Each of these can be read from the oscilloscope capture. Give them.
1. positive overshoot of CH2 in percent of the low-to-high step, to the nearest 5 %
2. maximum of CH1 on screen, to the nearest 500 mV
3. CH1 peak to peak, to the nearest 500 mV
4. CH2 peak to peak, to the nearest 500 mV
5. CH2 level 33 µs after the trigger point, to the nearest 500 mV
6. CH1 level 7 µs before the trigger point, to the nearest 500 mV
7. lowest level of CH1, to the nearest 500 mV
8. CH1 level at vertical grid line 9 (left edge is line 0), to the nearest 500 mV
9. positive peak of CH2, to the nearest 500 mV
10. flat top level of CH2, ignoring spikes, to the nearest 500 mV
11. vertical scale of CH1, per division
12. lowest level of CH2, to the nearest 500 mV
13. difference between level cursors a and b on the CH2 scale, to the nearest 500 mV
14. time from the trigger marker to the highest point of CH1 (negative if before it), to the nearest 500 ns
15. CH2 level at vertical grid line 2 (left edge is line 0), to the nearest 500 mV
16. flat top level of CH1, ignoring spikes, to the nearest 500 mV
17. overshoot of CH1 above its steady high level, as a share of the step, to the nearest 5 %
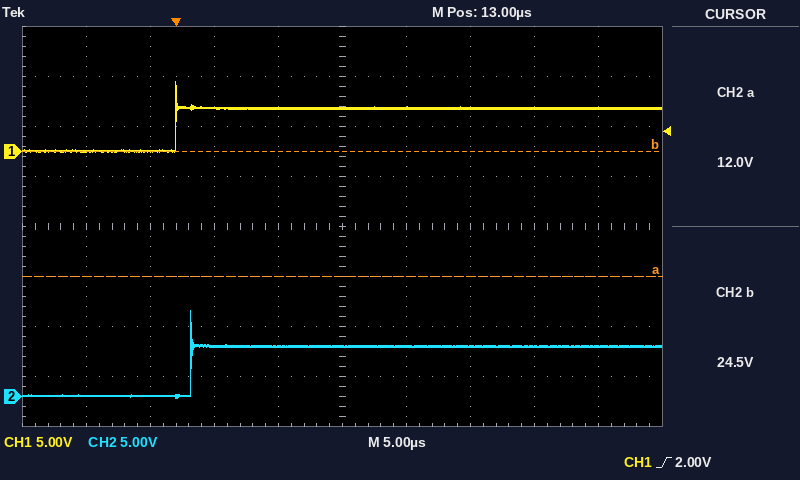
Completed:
70 %
7.0 V
7.0 V
8.5 V
5.0 V
0.0 V
0.0 V
4.5 V
8.5 V
5.0 V
5 V
0.0 V
12.5 V
0.0 µs
0.0 V
4.5 V
60 %
